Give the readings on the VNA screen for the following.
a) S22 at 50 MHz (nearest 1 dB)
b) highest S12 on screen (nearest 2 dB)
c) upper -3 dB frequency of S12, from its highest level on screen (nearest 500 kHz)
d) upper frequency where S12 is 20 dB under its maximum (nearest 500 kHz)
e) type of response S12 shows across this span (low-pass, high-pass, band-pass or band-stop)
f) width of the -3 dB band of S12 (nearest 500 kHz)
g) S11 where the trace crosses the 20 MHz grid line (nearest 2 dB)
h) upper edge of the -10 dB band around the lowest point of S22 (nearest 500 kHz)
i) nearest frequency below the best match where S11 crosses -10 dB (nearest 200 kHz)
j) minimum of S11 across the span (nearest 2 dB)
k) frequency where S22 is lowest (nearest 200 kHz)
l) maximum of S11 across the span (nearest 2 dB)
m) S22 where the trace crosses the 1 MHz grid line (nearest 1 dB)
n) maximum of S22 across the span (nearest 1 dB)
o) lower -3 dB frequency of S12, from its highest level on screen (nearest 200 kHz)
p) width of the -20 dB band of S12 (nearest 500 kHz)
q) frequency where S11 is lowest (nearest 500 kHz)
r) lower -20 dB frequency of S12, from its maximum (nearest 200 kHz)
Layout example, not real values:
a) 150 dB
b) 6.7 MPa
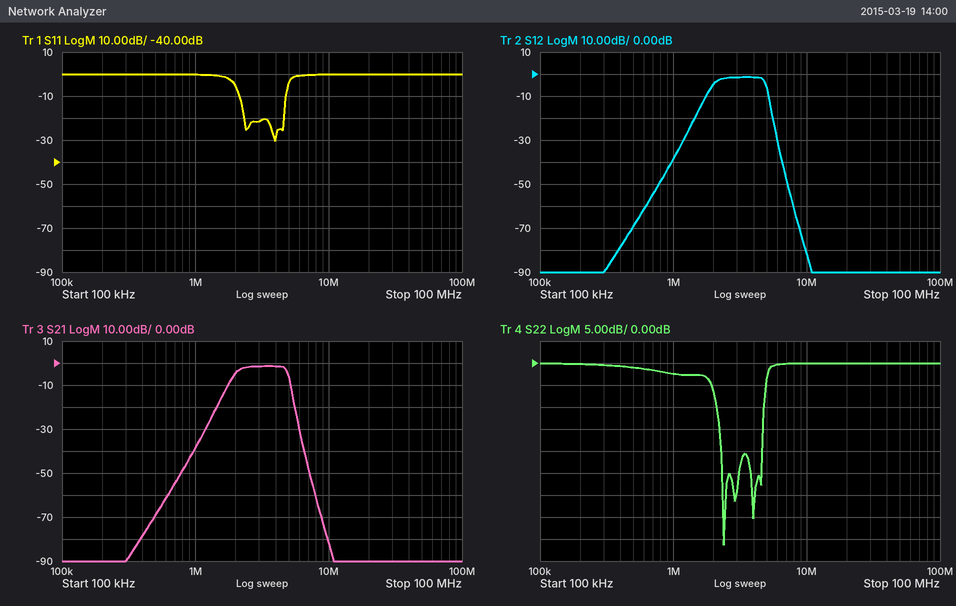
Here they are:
a) 0 dB
b) -2 dB
c) 5.0 MHz
d) 5.5 MHz
e) band-pass
f) 3.0 MHz
g) 0 dB
h) 5.0 MHz
i) 2.2 MHz
j) -30 dB
k) 2.4 MHz
l) 0 dB
m) -2 dB
n) 0 dB
o) 2.0 MHz
p) 4.0 MHz
q) 4.0 MHz
r) 1.4 MHz
